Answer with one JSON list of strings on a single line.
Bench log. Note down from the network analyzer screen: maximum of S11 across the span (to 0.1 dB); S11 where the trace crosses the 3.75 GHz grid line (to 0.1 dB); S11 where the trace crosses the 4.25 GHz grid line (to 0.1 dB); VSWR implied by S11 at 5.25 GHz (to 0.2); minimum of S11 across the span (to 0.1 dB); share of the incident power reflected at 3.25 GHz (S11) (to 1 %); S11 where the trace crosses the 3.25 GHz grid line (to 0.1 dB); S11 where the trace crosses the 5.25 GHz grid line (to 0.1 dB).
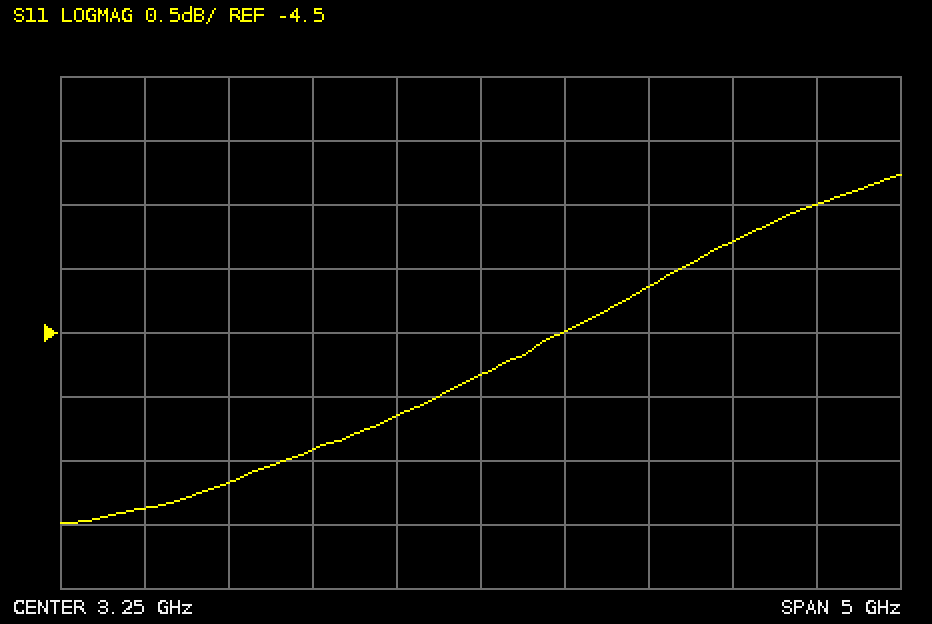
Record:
["-3.3 dB", "-4.5 dB", "-4.1 dB", "5.0", "-6.0 dB", "33 %", "-4.8 dB", "-3.5 dB"]
